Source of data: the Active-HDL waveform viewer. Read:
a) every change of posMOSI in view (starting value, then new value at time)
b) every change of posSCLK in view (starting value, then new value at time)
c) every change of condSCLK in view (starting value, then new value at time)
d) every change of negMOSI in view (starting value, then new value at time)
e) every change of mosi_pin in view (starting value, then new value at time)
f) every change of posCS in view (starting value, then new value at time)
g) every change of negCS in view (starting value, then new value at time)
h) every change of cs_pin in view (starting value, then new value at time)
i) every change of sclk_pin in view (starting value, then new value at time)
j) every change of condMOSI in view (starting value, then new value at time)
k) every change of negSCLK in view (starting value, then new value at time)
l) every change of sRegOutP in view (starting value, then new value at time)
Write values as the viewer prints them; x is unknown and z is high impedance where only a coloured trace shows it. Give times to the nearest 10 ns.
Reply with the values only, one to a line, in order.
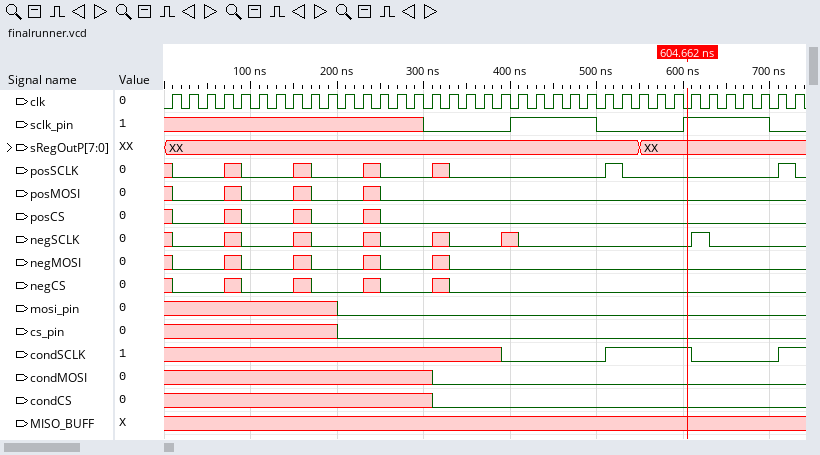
x, 0 at 10 ns, x at 70 ns, 0 at 90 ns, x at 150 ns, 0 at 170 ns, x at 230 ns, 0 at 250 ns
x, 0 at 10 ns, x at 70 ns, 0 at 90 ns, x at 150 ns, 0 at 170 ns, x at 230 ns, 0 at 250 ns, x at 310 ns, 0 at 330 ns, 1 at 510 ns, 0 at 530 ns, 1 at 710 ns, 0 at 730 ns
x, 0 at 390 ns, 1 at 510 ns, 0 at 610 ns, 1 at 710 ns
x, 0 at 10 ns, x at 70 ns, 0 at 90 ns, x at 150 ns, 0 at 170 ns, x at 230 ns, 0 at 250 ns, x at 310 ns, 0 at 330 ns
x, 0 at 200 ns
x, 0 at 10 ns, x at 70 ns, 0 at 90 ns, x at 150 ns, 0 at 170 ns, x at 230 ns, 0 at 250 ns
x, 0 at 10 ns, x at 70 ns, 0 at 90 ns, x at 150 ns, 0 at 170 ns, x at 230 ns, 0 at 250 ns, x at 310 ns, 0 at 330 ns
x, 0 at 200 ns
x, 0 at 300 ns, 1 at 400 ns, 0 at 500 ns, 1 at 600 ns, 0 at 700 ns
x, 0 at 310 ns
x, 0 at 10 ns, x at 70 ns, 0 at 90 ns, x at 150 ns, 0 at 170 ns, x at 230 ns, 0 at 250 ns, x at 310 ns, 0 at 330 ns, x at 390 ns, 0 at 410 ns, 1 at 610 ns, 0 at 630 ns
XX, XX at 550 ns
